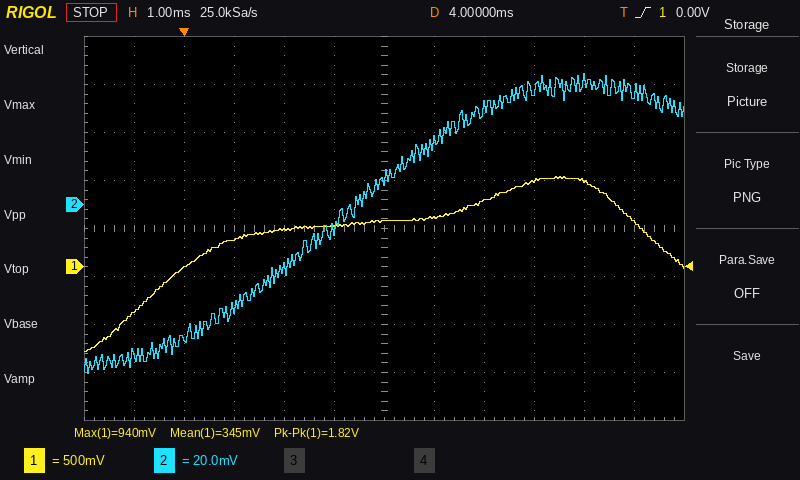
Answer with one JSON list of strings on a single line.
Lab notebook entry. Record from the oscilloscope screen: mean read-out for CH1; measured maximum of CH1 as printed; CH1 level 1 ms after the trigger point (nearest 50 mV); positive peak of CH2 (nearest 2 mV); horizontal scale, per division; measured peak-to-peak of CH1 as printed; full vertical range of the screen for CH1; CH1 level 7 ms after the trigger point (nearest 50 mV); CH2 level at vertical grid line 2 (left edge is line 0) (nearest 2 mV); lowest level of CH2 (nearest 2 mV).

["345 mV", "940 mV", "300 mV", "54 mV", "1 ms", "1.82 V", "4 V", "900 mV", "-56 mV", "-70 mV"]
